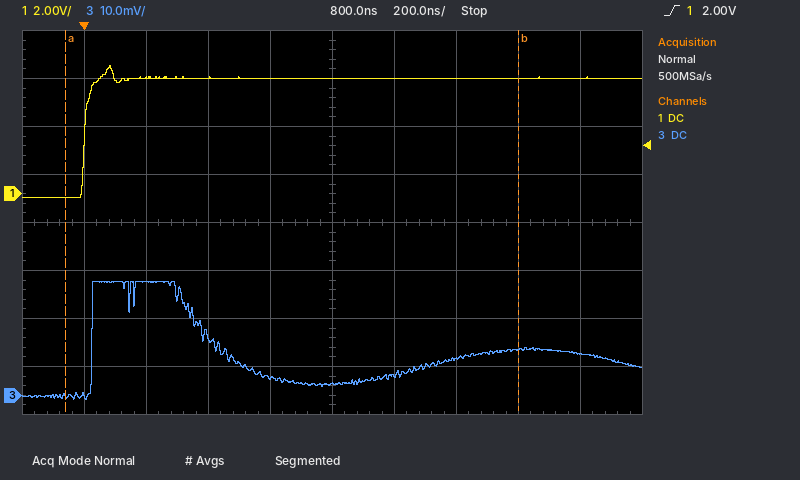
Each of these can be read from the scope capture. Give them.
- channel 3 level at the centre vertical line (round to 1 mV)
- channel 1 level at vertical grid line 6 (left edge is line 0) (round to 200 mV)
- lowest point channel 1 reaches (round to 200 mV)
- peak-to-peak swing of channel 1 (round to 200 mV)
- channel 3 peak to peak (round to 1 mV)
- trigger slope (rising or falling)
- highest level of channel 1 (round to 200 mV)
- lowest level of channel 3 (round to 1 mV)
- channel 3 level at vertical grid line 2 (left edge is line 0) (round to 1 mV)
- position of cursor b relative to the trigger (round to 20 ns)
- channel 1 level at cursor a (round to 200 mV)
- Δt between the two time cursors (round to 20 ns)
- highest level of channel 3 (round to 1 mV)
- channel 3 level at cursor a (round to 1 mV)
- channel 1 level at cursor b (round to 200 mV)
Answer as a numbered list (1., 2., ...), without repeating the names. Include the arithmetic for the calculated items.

1. 2 mV
2. 4.8 V
3. -200 mV
4. 5.4 V − (-200 mV) = 5.6 V
5. 24 mV − (-1 mV) = 25 mV
6. rising
7. 5.4 V
8. -1 mV
9. 24 mV
10. +1.40 µs
11. -200 mV
12. 1.46 µs
13. 24 mV
14. 0 mV
15. 4.8 V
